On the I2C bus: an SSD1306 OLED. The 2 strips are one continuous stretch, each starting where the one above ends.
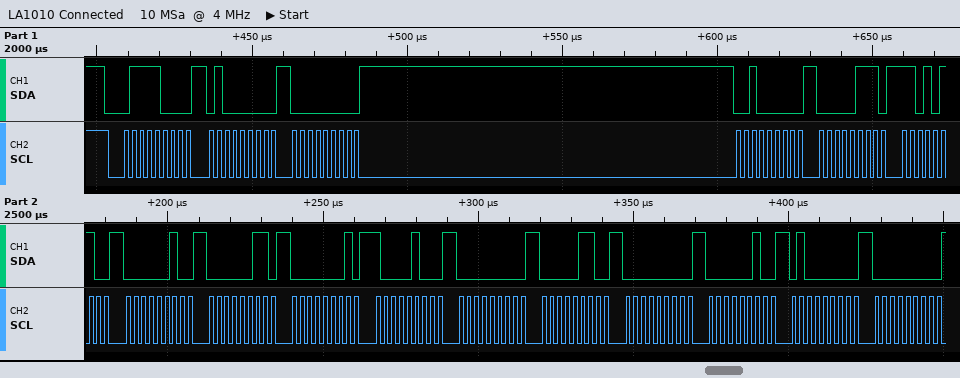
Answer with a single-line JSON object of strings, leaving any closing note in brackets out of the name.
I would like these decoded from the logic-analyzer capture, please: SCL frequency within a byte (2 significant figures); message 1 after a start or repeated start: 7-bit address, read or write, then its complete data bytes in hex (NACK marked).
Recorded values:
{"SCL frequency within a byte": "400 kHz", "message 1 after a start or repeated start: 7-bit address, read or write, then its complete data bytes in hex": "0x3C write: 40 00 20 07 D6 02 03 01 84 00 06 00 02 40 00"}
